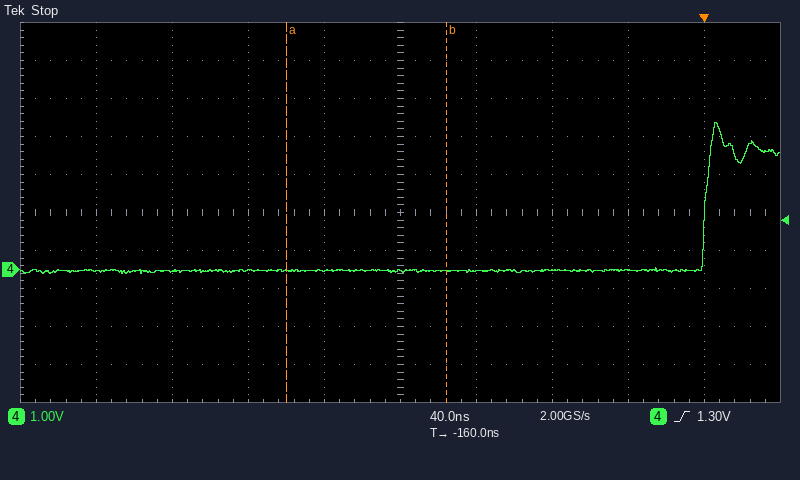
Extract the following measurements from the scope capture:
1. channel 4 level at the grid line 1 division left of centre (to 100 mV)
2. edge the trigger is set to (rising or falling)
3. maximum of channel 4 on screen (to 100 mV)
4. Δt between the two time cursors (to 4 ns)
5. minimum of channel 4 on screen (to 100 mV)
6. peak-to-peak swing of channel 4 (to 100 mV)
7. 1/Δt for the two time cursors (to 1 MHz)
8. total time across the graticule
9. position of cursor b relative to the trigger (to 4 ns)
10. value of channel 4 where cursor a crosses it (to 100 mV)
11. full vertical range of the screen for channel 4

0.0 V
rising
3.9 V
84 ns
-100 mV
4.0 V
12 MHz
400 ns
-136 ns
0.0 V
10 V
